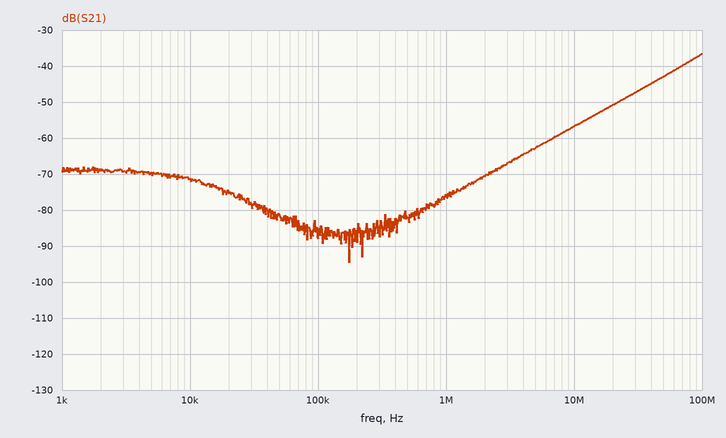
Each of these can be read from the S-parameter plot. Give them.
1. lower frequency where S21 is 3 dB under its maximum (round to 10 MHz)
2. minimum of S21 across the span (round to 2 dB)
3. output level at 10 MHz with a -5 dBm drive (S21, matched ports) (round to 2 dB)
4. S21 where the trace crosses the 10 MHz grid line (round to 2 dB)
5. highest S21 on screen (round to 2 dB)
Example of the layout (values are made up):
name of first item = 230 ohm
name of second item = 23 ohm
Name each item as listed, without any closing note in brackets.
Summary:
lower frequency where S21 is 3 dB under its maximum = 70 MHz
minimum of S21 across the span = -94 dB
output level at 10 MHz with a -5 dBm drive (S21, matched ports) = -62 dBm
S21 where the trace crosses the 10 MHz grid line = -56 dB
highest S21 on screen = -36 dB
